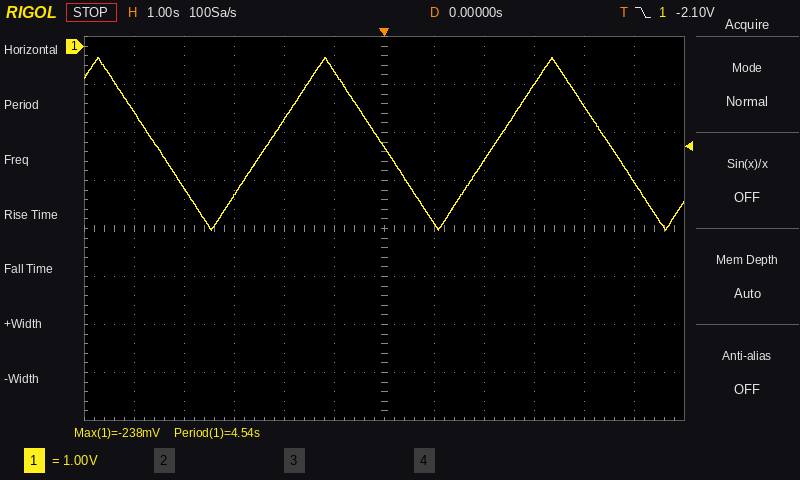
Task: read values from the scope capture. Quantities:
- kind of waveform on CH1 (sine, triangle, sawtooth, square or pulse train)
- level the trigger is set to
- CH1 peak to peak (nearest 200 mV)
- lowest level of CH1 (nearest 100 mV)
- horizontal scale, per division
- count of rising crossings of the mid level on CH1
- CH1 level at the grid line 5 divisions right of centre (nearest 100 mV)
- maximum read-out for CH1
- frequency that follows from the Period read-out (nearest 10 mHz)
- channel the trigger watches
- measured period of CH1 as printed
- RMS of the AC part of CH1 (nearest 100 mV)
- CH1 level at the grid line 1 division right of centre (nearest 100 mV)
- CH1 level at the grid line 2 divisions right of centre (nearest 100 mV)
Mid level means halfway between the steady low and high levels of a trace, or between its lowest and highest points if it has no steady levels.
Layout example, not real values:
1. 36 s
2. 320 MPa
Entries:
1. triangle
2. -2.10 V
3. 3.6 V
4. -3.8 V
5. 1 s
6. 2
7. -2.8 V
8. -238 mV
9. 220 mHz
10. CH1
11. 4.54 s
12. 1.0 V
13. -3.7 V
14. -2.4 V
